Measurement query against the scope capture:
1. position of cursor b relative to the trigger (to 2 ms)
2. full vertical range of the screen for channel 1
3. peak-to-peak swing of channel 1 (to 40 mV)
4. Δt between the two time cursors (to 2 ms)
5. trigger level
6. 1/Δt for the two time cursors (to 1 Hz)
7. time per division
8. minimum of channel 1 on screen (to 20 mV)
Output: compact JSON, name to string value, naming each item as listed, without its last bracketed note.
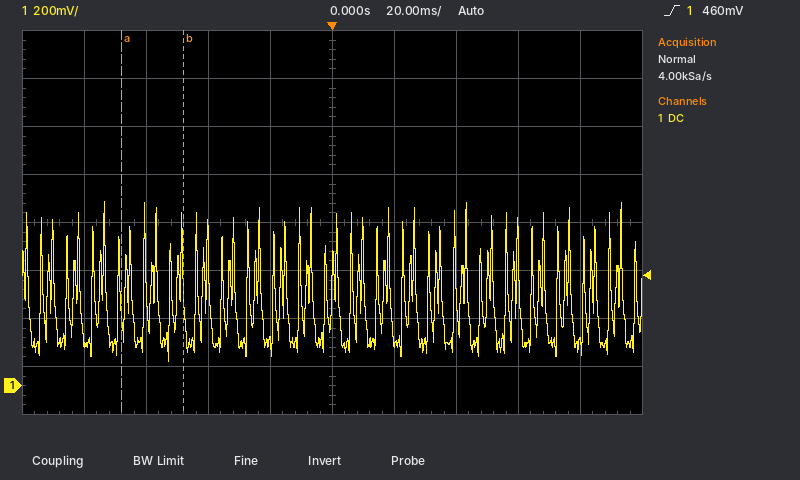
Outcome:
{"position of cursor b relative to the trigger": "-48 ms", "full vertical range of the screen for channel 1": "1.6 V", "peak-to-peak swing of channel 1": "680 mV", "Δt between the two time cursors": "20 ms", "trigger level": "460 mV", "1/Δt for the two time cursors": "50 Hz", "time per division": "20 ms", "minimum of channel 1 on screen": "100 mV"}
